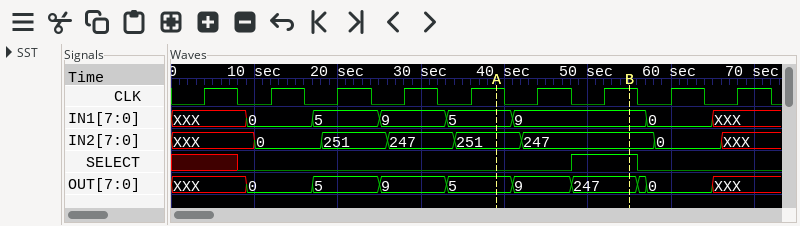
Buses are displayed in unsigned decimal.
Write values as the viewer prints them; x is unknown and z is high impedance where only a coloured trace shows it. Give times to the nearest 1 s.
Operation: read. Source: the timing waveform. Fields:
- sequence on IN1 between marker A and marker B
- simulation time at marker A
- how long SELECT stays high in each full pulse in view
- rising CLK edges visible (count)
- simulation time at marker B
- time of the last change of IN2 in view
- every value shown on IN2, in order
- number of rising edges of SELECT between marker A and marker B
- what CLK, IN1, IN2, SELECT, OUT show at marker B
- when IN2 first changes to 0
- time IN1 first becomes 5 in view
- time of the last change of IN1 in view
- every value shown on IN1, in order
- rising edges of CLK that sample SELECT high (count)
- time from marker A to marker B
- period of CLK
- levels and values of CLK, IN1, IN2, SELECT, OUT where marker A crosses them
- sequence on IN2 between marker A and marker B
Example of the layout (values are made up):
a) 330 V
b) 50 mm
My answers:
a) 5, 9
b) 39 s
c) 8 s
d) 9
e) 55 s
f) 66 s
g) XXX, 0, 251, 247, 251, 247, 0, XXX
h) 1
i) CLK=1, IN1=9, IN2=247, SELECT=1, OUT=247
j) 10 s
k) 17 s
l) 65 s
m) XXX, 0, 5, 9, 5, 9, 0, XXX
n) 1
o) 16 s
p) 8 s
q) CLK=1, IN1=5, IN2=251, SELECT=0, OUT=5
r) 251, 247
